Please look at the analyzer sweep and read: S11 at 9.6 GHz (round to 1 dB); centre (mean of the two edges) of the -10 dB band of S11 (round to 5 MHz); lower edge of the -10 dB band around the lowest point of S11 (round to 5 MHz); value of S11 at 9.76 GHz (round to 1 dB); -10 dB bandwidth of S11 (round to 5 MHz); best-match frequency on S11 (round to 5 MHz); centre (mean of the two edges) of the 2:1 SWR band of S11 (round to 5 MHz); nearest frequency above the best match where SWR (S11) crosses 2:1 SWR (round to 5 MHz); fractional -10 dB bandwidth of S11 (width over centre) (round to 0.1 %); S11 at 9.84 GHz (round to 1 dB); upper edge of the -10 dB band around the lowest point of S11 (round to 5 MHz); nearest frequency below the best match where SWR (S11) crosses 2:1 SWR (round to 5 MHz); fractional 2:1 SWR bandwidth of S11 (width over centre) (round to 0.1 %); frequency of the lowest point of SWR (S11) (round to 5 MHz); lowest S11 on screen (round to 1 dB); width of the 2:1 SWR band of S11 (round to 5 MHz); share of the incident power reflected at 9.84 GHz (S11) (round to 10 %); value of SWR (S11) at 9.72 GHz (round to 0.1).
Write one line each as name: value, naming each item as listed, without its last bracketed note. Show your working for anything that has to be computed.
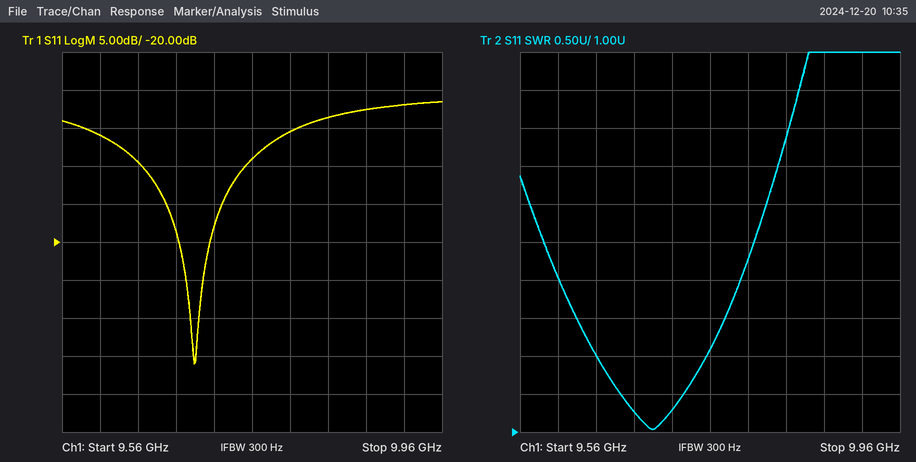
S11 at 9.6 GHz: -6 dB
centre (mean of the two edges) of the -10 dB band of S11: 9.700 GHz
lower edge of the -10 dB band around the lowest point of S11: 9.645 GHz
value of S11 at 9.76 GHz: -9 dB
-10 dB bandwidth of S11: 9.755 GHz − 9.645 GHz = 110 MHz
best-match frequency on S11: 9.700 GHz
centre (mean of the two edges) of the 2:1 SWR band of S11: 9.700 GHz
nearest frequency above the best match where SWR (S11) crosses 2:1 SWR: 9.755 GHz
fractional -10 dB bandwidth of S11 (width over centre): 110 MHz / 9.7 GHz ≈ 1.1 %
S11 at 9.84 GHz: -4 dB
upper edge of the -10 dB band around the lowest point of S11: 9.755 GHz
nearest frequency below the best match where SWR (S11) crosses 2:1 SWR: 9.640 GHz
fractional 2:1 SWR bandwidth of S11 (width over centre): 115 MHz / 9.6975 GHz ≈ 1.2 %
frequency of the lowest point of SWR (S11): 9.700 GHz
lowest S11 on screen: -36 dB
width of the 2:1 SWR band of S11: 9.755 GHz − 9.640 GHz = 115 MHz
share of the incident power reflected at 9.84 GHz (S11): 10^(-4/10) ≈ 40 %
value of SWR (S11) at 9.72 GHz: 1.3
